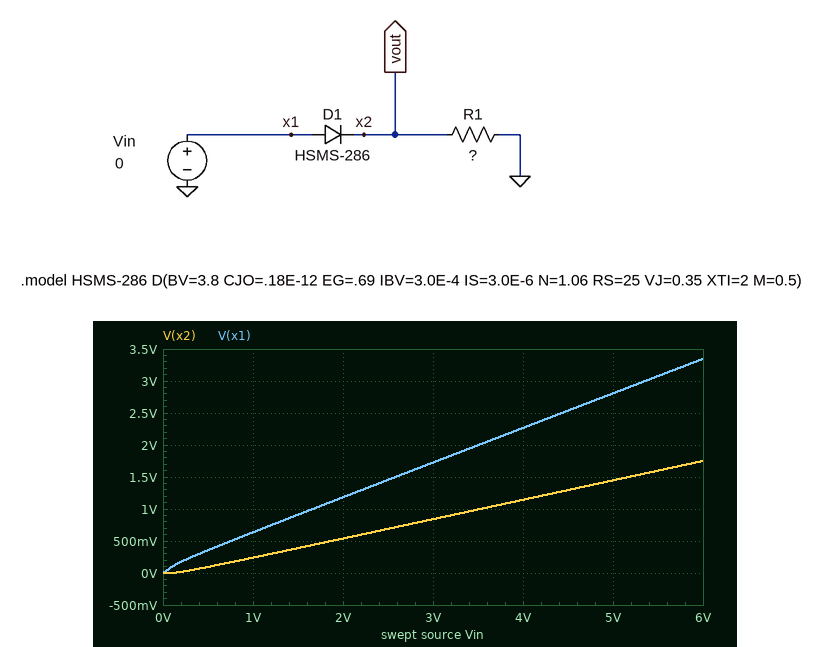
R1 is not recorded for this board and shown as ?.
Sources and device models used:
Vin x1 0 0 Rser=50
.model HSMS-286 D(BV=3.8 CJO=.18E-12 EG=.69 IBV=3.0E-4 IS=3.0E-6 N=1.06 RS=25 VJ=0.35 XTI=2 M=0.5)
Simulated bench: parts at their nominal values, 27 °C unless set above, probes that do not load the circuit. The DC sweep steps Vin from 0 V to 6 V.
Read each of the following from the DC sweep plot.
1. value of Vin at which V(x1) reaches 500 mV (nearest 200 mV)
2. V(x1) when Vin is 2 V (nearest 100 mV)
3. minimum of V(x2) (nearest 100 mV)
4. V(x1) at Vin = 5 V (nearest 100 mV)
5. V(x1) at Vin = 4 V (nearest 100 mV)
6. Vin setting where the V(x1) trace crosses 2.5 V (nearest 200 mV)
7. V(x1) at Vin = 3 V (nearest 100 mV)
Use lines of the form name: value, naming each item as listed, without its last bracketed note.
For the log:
value of Vin at which V(x1) reaches 500 mV: 800 mV
V(x1) when Vin is 2 V: 1.2 V
minimum of V(x2): 0 V
V(x1) at Vin = 5 V: 2.8 V
V(x1) at Vin = 4 V: 2.3 V
Vin setting where the V(x1) trace crosses 2.5 V: 4.4 V
V(x1) at Vin = 3 V: 1.7 V
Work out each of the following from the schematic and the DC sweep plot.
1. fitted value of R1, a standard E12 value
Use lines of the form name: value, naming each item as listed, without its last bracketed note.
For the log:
fitted value of R1, a standard E12 value: 33 Ω
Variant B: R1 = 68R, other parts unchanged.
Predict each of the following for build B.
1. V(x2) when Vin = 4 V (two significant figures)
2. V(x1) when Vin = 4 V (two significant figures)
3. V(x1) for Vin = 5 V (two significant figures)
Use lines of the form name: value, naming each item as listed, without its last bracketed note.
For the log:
V(x2) when Vin = 4 V: 1.8 V
V(x1) when Vin = 4 V: 2.7 V
V(x1) for Vin = 5 V: 3.3 V
